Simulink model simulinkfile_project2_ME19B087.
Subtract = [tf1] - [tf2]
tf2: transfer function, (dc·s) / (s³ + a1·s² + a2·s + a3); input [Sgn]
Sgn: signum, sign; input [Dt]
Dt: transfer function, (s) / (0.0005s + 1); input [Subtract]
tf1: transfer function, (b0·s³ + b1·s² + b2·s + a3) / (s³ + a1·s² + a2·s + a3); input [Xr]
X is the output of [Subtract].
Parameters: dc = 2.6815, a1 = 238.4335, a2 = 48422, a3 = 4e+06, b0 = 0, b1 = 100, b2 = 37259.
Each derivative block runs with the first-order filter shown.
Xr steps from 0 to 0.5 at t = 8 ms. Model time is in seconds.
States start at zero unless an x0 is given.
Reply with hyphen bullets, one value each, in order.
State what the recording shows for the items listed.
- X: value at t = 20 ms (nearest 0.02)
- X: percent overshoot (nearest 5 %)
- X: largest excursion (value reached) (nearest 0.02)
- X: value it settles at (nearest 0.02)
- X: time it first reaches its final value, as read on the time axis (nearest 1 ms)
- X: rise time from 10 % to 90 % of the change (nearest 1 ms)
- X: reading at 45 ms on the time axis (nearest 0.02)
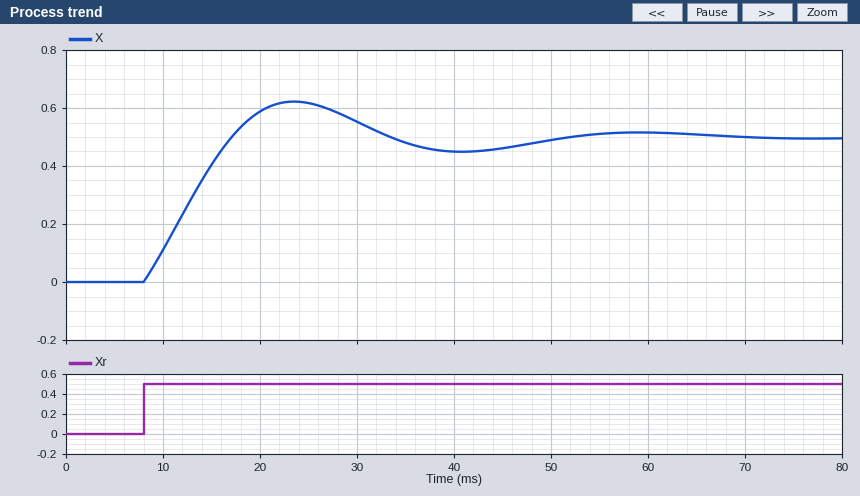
- 0.58
- 25 %
- 0.62
- 0.50
- 17 ms
- 7 ms
- 0.46
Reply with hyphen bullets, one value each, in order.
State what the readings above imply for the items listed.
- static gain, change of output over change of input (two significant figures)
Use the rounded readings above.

- 1.0
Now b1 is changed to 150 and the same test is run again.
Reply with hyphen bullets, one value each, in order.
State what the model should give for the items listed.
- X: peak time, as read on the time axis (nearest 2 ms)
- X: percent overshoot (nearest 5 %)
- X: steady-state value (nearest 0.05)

- 22 ms
- 20 %
- 0.50
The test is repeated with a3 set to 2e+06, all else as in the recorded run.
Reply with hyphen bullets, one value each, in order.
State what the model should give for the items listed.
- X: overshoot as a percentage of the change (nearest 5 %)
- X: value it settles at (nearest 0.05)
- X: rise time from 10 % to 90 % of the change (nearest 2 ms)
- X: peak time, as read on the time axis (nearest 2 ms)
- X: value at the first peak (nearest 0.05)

- 10 %
- 0.50
- 8 ms
- 24 ms
- 0.55
